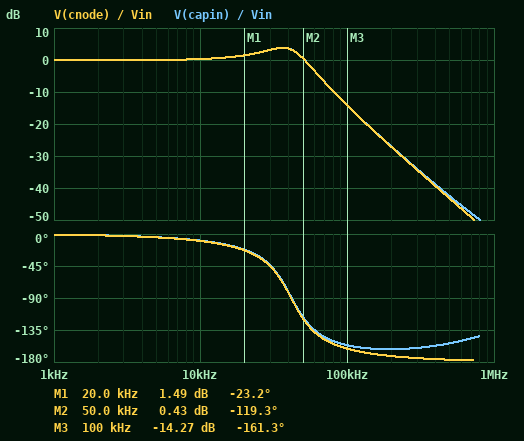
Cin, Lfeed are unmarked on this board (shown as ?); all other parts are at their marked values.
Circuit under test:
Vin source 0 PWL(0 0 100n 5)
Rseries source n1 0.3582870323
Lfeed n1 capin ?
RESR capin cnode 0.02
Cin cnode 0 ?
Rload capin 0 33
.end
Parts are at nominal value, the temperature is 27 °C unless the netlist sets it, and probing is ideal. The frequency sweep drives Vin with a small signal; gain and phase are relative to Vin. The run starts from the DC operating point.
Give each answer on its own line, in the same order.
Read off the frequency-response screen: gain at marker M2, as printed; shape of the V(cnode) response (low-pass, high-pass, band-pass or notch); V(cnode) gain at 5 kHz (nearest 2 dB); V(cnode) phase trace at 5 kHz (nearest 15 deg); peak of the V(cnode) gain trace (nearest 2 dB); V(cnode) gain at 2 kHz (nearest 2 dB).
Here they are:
0.43 dB
low-pass
0 dB
0 deg
4 dB
0 dB
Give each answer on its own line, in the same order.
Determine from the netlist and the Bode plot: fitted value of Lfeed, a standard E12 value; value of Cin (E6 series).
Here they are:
2.2 µH
6.8 µF
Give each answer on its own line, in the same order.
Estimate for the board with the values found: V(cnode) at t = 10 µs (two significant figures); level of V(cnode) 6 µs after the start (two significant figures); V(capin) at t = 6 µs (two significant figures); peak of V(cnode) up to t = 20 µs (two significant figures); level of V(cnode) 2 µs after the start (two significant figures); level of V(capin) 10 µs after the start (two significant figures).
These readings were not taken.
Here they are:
6.0 V
3.6 V
3.7 V
6.5 V
560 mV
6.1 V
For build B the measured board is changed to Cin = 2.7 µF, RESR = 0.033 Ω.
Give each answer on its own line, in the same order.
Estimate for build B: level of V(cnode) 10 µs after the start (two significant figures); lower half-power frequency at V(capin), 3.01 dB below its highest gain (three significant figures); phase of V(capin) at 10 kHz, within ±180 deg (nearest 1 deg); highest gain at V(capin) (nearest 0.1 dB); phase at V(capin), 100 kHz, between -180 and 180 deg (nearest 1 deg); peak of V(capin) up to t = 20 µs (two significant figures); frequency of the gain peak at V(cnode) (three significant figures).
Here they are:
6.6 V
44.0 kHz
-4 deg
6.9 dB
-149 deg
7.3 V
62.1 kHz
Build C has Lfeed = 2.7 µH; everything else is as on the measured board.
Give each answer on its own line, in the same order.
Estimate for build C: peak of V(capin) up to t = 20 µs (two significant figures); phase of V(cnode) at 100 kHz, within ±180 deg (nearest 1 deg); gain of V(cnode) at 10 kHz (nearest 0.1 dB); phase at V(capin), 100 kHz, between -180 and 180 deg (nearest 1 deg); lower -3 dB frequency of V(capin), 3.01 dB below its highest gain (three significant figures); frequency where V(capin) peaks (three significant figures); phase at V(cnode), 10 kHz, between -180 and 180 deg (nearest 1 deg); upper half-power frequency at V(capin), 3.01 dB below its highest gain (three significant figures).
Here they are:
6.7 V
-165 deg
0.4 dB
-160 deg
17.7 kHz
33.6 kHz
-10 deg
44.1 kHz
